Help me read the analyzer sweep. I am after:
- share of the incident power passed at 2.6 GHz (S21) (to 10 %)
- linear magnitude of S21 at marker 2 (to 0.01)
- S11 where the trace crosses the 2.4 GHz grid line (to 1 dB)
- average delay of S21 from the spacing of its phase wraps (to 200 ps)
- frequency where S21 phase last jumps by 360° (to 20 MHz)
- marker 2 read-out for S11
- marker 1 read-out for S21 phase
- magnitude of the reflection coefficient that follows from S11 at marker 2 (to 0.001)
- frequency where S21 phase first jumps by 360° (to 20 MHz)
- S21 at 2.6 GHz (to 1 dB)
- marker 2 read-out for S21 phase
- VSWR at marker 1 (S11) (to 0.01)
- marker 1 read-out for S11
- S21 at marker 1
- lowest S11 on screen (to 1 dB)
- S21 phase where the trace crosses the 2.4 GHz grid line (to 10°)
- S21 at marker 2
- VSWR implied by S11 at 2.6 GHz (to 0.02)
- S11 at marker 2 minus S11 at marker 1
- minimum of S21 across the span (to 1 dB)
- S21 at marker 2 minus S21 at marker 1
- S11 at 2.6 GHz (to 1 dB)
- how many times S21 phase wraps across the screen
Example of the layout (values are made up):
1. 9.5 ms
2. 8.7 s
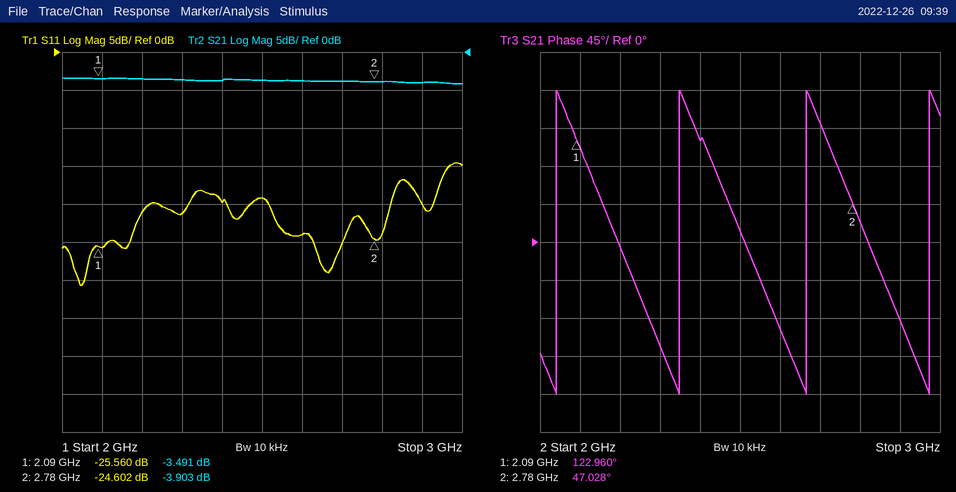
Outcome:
1. 40 %
2. 0.64
3. -20 dB
4. 3.2 ns
5. 2.98 GHz
6. -24.602 dB
7. 122.960°
8. 0.059
9. 2.04 GHz
10. -4 dB
11. 47.028°
12. 1.11
13. -25.560 dB
14. -3.491 dB
15. -31 dB
16. 120°
17. -3.903 dB
18. 1.14
19. 0.958 dB
20. -4 dB
21. -0.412 dB
22. -24 dB
23. 4
